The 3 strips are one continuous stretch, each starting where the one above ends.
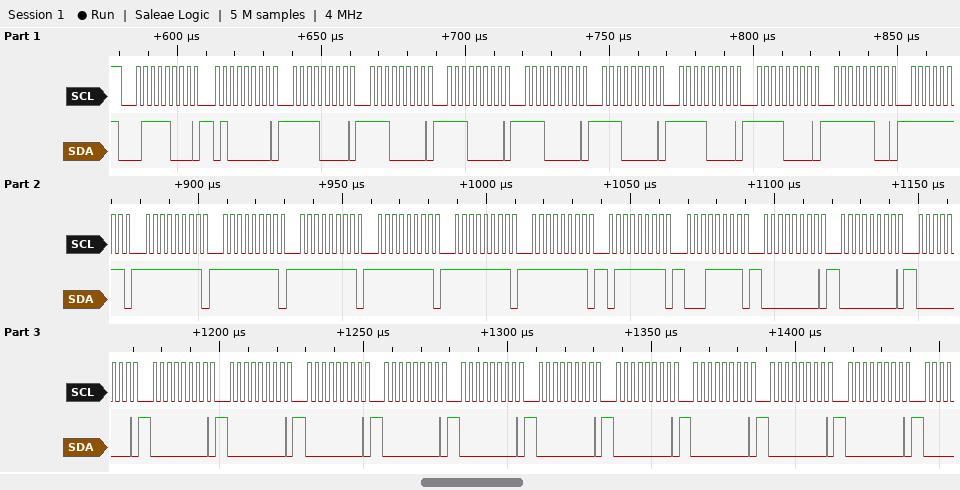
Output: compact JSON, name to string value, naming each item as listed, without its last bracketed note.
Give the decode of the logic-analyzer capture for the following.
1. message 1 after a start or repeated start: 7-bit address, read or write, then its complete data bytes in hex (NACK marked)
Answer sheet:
{"message 1 after a start or repeated start: 7-bit address, read or write, then its complete data bytes in hex": "0x3C write: 40 F0 E0 E0 E0 E0 F0 F0 FC FF FF FF FF FF FF FF 7F 1F 00 00 00 00 00 00 00 00 00 00 00 00 00"}
